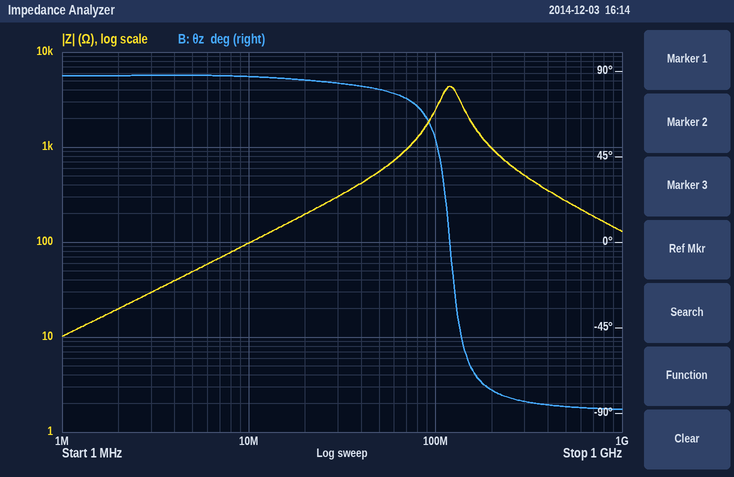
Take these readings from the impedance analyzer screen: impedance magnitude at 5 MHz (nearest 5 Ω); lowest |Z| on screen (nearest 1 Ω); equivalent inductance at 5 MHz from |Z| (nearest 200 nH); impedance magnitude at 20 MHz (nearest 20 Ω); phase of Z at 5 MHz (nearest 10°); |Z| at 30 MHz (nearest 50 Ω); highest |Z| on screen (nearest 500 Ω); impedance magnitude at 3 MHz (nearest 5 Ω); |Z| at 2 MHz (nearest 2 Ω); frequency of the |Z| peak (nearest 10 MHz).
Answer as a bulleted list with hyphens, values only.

- 50 Ω
- 10 Ω
- 1.6 µH
- 200 Ω
- 90°
- 300 Ω
- 4.5 kΩ
- 30 Ω
- 20 Ω
- 120 MHz
